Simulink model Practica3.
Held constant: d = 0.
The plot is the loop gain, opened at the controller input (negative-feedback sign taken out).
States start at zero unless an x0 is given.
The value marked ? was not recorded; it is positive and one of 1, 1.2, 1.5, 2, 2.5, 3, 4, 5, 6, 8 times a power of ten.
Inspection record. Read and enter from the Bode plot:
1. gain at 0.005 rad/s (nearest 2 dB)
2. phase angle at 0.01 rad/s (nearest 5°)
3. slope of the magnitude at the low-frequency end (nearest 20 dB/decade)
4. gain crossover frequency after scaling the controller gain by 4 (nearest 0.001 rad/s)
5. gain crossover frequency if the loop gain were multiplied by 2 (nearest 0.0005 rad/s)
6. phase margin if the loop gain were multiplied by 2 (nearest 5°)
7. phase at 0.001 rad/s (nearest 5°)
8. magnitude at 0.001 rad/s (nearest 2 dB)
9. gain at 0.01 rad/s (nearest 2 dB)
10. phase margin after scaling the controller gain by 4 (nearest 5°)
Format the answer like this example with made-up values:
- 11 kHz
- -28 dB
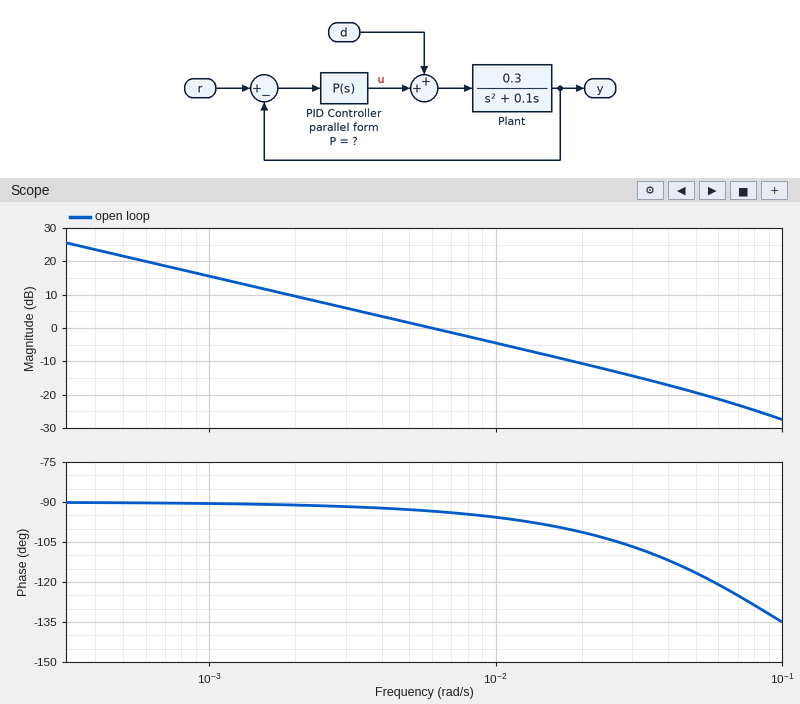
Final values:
- 2 dB
- -95°
- -20 dB/decade
- 0.023 rad/s
- 0.0120 rad/s
- 85°
- -90°
- 16 dB
- -4 dB
- 75°
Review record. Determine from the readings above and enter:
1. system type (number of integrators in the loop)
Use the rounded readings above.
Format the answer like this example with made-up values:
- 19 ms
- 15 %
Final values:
- 1
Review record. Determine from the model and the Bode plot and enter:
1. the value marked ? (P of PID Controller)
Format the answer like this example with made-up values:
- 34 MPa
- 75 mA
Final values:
- 0.002
